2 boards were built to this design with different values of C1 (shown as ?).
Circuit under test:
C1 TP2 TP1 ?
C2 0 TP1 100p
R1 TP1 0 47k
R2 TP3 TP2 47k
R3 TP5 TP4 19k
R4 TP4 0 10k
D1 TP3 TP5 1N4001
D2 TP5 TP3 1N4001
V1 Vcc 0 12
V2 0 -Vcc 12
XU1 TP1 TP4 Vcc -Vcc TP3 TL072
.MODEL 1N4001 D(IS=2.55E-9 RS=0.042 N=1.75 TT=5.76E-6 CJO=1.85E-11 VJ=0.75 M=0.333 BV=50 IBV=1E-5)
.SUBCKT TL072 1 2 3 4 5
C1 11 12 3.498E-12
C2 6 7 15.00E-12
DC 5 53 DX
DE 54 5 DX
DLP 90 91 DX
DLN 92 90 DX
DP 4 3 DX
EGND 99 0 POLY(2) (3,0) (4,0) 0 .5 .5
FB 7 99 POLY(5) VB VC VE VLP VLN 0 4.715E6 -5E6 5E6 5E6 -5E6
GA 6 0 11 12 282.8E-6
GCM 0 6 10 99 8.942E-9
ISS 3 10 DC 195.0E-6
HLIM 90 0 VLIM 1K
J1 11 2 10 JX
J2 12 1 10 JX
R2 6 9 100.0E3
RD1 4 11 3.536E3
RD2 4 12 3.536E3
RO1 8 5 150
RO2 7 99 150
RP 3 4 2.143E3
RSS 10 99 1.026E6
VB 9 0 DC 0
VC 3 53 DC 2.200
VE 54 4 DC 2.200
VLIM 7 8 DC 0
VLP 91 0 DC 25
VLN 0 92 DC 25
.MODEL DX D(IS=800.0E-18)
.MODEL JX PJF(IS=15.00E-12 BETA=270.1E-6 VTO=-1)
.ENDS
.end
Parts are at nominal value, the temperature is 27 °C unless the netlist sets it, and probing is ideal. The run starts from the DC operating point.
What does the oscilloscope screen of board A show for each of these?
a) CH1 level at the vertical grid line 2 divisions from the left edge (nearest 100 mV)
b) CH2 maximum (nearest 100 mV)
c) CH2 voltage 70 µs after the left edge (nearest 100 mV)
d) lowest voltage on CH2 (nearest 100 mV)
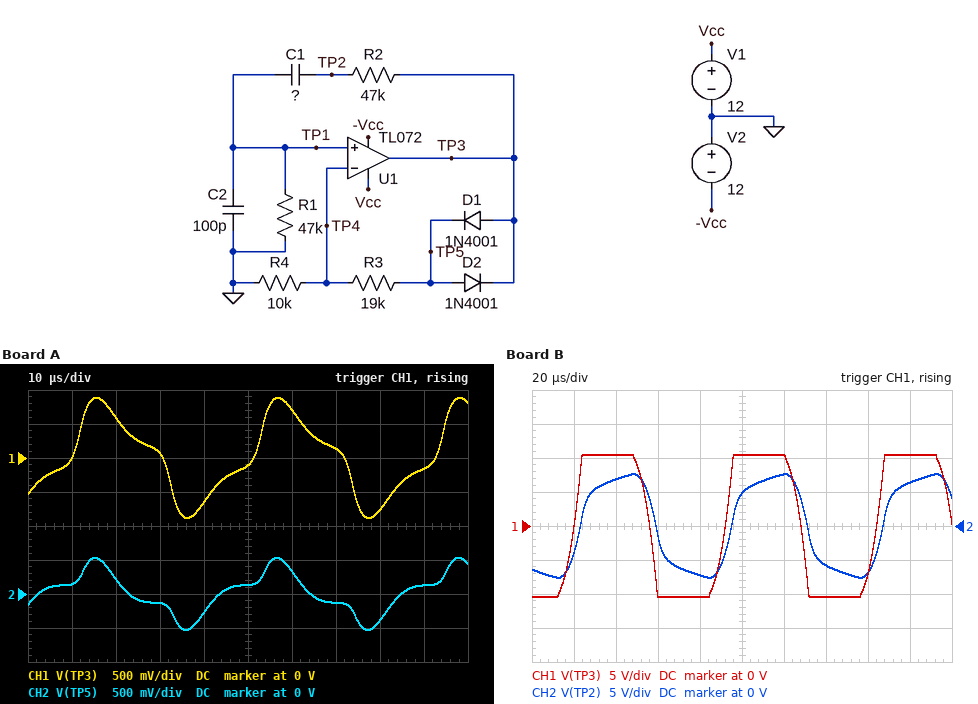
600 mV
500 mV
-100 mV
-500 mV
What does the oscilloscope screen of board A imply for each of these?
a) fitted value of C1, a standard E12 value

39 pF
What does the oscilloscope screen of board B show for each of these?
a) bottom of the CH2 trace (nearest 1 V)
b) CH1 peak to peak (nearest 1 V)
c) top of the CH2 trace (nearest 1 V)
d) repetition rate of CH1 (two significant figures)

-8 V
21 V
8 V
14 kHz
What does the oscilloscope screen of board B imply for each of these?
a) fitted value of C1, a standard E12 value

330 pF
